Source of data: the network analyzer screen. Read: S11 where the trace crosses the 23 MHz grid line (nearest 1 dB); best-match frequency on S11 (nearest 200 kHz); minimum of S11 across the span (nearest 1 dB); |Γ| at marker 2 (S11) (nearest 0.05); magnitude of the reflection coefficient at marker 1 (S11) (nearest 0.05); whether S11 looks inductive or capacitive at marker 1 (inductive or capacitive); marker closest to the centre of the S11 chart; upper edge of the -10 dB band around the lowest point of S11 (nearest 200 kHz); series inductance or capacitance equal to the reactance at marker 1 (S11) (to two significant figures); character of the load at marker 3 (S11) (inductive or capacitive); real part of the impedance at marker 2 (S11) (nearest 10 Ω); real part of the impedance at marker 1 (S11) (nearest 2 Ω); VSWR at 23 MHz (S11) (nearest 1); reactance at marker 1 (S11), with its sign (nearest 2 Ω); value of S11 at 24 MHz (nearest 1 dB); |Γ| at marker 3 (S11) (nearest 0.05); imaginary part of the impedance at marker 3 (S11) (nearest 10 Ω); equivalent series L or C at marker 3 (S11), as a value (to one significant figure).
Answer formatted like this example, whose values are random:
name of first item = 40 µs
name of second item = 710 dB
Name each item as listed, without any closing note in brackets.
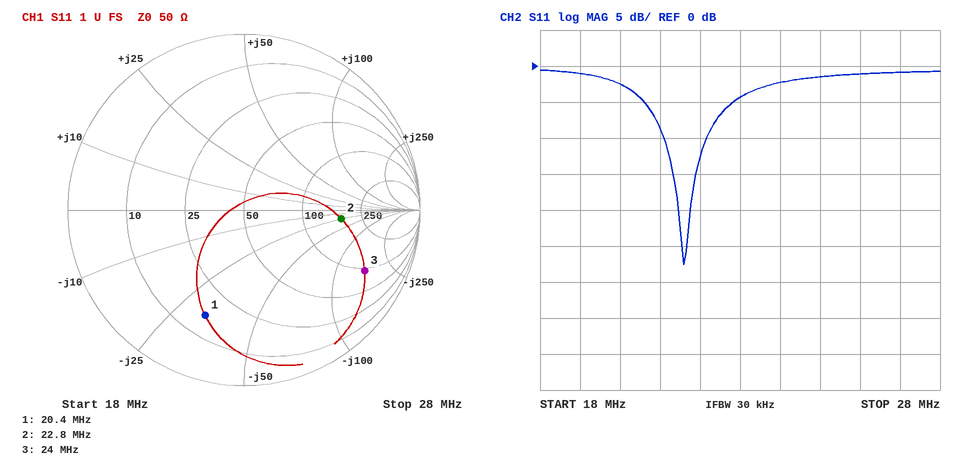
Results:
S11 where the trace crosses the 23 MHz grid line = -4 dB
best-match frequency on S11 = 21.6 MHz
minimum of S11 across the span = -28 dB
|Γ| at marker 2 (S11) = 0.55
magnitude of the reflection coefficient at marker 1 (S11) = 0.65
whether S11 looks inductive or capacitive at marker 1 = capacitive
marker closest to the centre of the S11 chart = marker 2
upper edge of the -10 dB band around the lowest point of S11 = 22.2 MHz
series inductance or capacitance equal to the reactance at marker 1 (S11) = 240 pF
character of the load at marker 3 (S11) = capacitive
real part of the impedance at marker 2 (S11) = 170 Ω
real part of the impedance at marker 1 (S11) = 16 Ω
VSWR at 23 MHz (S11) = 4
reactance at marker 1 (S11), with its sign = -32 Ω
value of S11 at 24 MHz = -2 dB
|Γ| at marker 3 (S11) = 0.75
imaginary part of the impedance at marker 3 (S11) = -160 Ω
equivalent series L or C at marker 3 (S11), as a value = 40 pF
